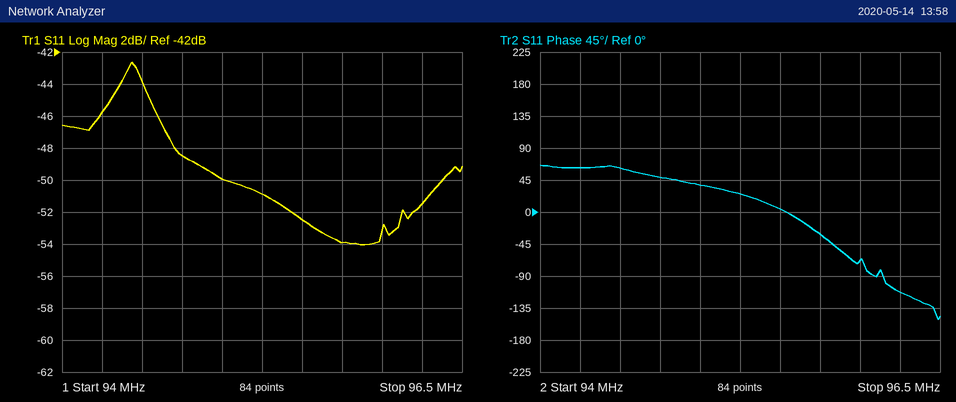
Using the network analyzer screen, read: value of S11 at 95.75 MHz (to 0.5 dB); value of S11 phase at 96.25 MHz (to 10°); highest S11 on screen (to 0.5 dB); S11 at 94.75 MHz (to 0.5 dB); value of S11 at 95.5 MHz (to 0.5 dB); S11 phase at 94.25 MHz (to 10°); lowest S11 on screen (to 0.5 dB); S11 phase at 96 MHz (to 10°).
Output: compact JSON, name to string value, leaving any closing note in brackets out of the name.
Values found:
{"value of S11 at 95.75 MHz": "-54.0 dB", "value of S11 phase at 96.25 MHz": "-110°", "highest S11 on screen": "-42.5 dB", "S11 at 94.75 MHz": "-48.5 dB", "value of S11 at 95.5 MHz": "-52.5 dB", "S11 phase at 94.25 MHz": "60°", "lowest S11 on screen": "-54.0 dB", "S11 phase at 96 MHz": "-70°"}
